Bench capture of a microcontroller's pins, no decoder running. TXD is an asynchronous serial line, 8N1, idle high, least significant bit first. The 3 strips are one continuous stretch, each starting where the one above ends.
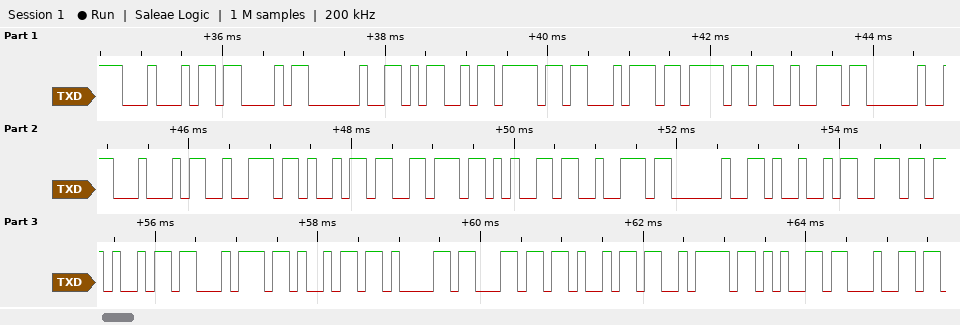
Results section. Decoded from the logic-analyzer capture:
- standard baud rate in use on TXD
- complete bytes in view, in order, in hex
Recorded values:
9600 baud
0x44 0x43 0x20 0x4D 0x6F 0x74 0x6F 0x72 0x20 0x44 0x72 0x69 0x76 0x65 0x72 0x20 0x49 0x6E 0x69 0x74 0x69 0x61 0x6C 0x69 0x7A 0x65 0x64
